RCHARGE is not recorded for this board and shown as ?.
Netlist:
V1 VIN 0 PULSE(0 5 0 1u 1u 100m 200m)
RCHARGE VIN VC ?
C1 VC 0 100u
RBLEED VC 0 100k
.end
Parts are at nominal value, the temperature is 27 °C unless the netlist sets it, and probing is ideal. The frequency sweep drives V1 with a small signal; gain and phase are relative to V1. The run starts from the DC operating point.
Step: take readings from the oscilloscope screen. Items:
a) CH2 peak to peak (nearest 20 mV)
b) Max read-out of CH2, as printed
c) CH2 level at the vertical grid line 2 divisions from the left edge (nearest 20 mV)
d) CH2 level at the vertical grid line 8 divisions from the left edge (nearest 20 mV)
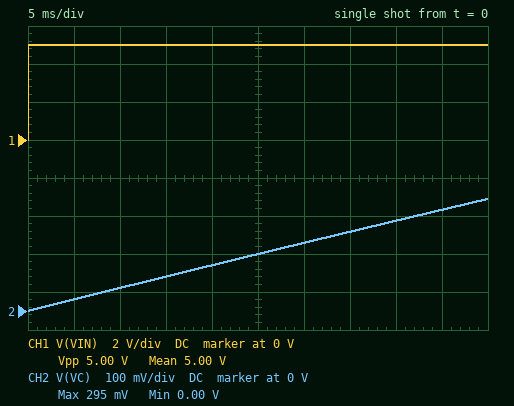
300 mV
295 mV
60 mV
240 mV
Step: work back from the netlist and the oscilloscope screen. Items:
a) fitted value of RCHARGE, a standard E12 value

8.2 kΩ
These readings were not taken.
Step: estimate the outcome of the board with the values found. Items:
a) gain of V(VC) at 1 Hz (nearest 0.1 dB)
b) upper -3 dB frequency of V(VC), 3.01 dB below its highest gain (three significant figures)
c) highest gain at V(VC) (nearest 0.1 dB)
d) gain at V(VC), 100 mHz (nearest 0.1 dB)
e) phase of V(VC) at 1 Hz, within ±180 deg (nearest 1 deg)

-14.4 dB
210 mHz
-0.7 dB
-1.6 dB
-78 deg
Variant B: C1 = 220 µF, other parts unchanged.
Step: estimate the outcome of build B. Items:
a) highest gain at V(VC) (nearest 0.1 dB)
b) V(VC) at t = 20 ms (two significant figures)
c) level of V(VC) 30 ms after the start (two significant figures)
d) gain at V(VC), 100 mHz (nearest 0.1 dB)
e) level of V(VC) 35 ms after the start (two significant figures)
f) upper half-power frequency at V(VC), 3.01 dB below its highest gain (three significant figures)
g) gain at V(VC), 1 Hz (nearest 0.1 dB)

-0.7 dB
55 mV
82 mV
-3.9 dB
96 mV
95.5 mHz
-21.1 dB
